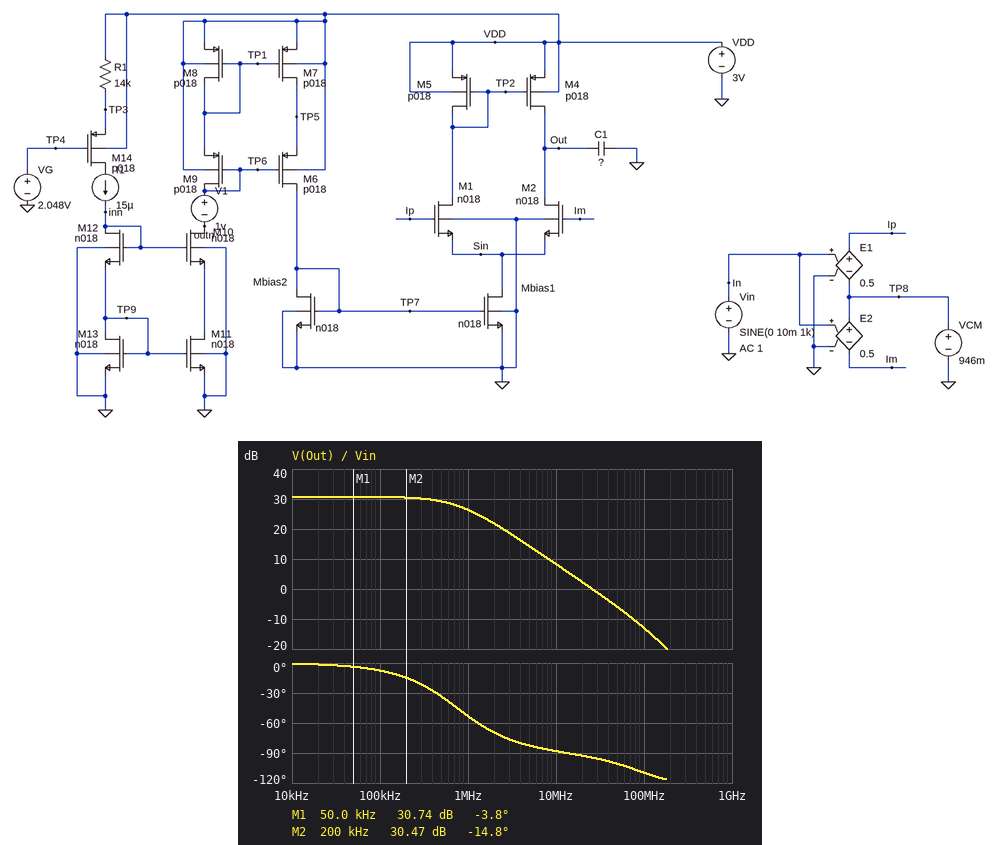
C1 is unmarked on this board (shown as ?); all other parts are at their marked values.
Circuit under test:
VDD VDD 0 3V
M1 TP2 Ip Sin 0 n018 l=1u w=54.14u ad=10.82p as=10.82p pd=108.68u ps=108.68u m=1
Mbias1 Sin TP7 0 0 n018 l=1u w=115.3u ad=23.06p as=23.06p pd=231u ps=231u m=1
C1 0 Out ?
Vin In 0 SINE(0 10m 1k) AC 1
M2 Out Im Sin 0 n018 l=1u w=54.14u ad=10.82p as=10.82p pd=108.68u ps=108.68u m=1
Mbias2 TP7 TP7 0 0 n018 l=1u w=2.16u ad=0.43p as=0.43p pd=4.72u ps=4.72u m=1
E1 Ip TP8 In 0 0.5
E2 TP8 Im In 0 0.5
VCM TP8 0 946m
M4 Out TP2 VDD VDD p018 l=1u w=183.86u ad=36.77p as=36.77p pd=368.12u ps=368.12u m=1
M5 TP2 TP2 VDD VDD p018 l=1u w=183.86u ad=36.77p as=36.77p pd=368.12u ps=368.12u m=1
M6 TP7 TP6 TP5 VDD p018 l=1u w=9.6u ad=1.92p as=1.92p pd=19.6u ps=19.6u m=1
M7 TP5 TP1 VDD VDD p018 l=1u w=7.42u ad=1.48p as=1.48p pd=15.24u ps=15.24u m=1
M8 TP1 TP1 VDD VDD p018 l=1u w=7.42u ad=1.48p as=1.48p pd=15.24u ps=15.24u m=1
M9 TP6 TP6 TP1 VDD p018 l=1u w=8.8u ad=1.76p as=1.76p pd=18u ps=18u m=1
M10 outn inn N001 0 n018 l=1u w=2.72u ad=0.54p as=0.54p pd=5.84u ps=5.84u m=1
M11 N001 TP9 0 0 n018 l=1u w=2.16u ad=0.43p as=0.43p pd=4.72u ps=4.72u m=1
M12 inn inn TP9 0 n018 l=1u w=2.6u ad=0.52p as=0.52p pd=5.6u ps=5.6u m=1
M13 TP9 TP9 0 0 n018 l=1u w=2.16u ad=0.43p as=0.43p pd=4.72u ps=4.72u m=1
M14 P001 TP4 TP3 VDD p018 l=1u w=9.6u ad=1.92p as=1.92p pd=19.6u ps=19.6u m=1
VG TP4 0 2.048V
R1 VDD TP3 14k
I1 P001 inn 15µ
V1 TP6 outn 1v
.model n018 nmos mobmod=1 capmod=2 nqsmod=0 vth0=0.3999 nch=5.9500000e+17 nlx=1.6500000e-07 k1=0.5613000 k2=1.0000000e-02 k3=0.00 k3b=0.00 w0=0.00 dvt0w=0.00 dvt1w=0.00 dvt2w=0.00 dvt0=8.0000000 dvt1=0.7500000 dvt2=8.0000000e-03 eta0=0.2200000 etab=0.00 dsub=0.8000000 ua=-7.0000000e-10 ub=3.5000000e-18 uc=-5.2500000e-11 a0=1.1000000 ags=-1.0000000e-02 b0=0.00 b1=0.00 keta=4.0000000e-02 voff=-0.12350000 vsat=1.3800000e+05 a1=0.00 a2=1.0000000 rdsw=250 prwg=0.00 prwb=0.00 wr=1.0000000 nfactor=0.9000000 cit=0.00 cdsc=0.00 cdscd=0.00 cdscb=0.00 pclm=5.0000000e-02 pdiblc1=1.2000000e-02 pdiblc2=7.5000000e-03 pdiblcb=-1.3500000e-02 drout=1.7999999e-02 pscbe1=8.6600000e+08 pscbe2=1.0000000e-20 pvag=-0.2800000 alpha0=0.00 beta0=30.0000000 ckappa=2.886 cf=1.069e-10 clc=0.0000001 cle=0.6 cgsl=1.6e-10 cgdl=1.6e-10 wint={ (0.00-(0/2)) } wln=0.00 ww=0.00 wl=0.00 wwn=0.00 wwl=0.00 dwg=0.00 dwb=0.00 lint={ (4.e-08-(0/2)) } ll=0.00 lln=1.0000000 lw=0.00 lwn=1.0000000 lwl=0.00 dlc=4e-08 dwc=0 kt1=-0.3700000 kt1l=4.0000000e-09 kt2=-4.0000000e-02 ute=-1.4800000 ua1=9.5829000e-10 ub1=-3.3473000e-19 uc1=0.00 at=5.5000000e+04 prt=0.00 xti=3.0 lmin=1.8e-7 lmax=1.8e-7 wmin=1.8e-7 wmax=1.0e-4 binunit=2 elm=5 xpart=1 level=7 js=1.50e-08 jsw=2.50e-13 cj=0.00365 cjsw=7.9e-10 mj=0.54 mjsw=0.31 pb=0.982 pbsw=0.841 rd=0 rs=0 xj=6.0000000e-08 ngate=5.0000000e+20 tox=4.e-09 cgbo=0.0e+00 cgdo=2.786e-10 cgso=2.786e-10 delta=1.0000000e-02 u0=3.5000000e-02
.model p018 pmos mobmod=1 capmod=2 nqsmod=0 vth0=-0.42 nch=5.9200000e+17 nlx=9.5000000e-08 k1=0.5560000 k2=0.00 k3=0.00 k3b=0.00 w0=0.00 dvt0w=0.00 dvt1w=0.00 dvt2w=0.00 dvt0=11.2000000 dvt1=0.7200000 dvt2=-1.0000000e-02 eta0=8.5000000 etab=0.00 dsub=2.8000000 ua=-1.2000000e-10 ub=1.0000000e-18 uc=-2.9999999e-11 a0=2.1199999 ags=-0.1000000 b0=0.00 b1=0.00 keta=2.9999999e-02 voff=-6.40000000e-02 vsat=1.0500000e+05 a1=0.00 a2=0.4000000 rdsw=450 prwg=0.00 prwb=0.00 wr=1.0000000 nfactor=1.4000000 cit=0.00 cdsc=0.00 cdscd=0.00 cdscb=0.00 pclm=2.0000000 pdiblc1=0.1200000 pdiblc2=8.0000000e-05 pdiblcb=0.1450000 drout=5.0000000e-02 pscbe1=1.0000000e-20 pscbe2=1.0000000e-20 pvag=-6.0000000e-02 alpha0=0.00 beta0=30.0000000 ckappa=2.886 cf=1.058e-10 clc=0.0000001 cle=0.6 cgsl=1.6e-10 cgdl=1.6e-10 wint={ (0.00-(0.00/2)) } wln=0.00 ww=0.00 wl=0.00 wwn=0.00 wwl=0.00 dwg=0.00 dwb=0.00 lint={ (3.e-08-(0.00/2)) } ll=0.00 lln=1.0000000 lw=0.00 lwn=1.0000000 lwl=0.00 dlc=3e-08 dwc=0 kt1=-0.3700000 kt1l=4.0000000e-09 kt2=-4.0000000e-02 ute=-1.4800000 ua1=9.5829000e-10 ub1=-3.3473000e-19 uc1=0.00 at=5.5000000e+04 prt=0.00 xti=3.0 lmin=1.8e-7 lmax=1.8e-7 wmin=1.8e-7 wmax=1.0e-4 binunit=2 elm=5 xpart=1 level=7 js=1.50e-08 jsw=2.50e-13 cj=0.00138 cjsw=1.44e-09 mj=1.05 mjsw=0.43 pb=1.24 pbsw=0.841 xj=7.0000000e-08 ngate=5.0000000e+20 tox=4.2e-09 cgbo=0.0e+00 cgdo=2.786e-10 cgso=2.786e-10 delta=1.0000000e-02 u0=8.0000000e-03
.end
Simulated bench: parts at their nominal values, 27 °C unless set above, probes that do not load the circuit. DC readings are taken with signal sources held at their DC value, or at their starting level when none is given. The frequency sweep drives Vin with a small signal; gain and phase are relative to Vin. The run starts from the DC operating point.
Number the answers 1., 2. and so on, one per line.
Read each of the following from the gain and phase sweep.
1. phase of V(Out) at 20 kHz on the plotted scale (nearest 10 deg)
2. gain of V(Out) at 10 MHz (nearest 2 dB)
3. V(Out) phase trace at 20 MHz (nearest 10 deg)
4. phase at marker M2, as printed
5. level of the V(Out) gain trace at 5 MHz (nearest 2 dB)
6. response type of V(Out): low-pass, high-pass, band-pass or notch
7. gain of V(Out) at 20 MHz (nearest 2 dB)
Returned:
1. 0 deg
2. 8 dB
3. -90 deg
4. -14.8 deg
5. 14 dB
6. low-pass
7. 2 dB
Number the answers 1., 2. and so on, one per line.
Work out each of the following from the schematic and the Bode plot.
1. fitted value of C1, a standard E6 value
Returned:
1. 15 pF
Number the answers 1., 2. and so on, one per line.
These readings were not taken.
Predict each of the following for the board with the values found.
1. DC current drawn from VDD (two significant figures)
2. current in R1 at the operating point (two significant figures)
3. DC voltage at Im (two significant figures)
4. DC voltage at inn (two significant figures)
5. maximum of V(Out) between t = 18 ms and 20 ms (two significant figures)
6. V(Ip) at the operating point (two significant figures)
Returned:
1. 1.0 mA
2. 15 µA
3. 950 mV
4. 1.5 V
5. 2.5 V
6. 950 mV
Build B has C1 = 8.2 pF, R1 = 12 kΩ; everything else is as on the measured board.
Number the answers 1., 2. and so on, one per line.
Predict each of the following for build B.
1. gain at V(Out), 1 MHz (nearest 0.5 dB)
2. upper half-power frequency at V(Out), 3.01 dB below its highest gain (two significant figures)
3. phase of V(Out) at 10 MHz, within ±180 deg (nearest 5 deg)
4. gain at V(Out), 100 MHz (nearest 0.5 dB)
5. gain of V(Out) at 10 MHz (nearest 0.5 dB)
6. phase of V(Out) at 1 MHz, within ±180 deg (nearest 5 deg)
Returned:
1. 29.0 dB
2. 1.3 MHz
3. -85 deg
4. -8.0 dB
5. 13.0 dB
6. -35 deg
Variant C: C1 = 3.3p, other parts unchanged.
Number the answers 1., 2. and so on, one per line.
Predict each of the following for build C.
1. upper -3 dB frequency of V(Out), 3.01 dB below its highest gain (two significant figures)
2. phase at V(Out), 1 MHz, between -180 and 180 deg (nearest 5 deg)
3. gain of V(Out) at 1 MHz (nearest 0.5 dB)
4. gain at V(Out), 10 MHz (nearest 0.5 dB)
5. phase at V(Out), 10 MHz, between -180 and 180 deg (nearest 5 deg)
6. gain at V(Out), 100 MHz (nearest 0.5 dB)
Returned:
1. 3.0 MHz
2. -20 deg
3. 30.5 dB
4. 20.0 dB
5. -75 deg
6. -1.0 dB
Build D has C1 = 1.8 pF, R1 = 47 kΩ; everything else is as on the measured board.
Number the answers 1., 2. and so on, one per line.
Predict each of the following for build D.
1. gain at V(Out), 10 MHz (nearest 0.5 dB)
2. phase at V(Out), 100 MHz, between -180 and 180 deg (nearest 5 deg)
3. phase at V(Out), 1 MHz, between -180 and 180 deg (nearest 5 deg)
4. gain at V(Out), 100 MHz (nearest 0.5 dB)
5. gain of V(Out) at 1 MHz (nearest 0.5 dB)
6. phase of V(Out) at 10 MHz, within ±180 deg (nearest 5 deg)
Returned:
1. 23.5 dB
2. -105 deg
3. -10 deg
4. 3.0 dB
5. 30.5 dB
6. -65 deg
